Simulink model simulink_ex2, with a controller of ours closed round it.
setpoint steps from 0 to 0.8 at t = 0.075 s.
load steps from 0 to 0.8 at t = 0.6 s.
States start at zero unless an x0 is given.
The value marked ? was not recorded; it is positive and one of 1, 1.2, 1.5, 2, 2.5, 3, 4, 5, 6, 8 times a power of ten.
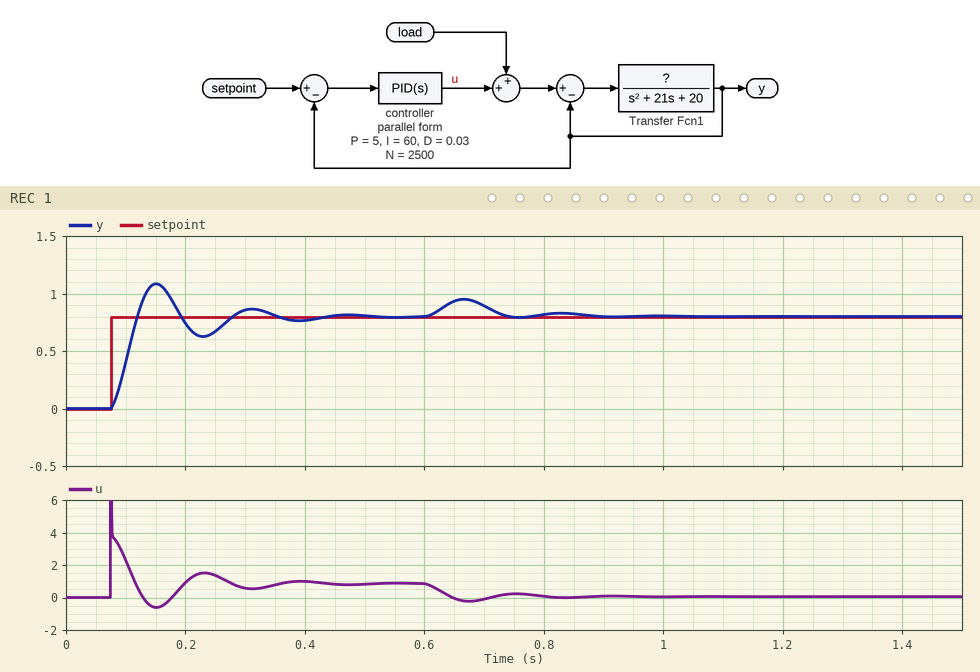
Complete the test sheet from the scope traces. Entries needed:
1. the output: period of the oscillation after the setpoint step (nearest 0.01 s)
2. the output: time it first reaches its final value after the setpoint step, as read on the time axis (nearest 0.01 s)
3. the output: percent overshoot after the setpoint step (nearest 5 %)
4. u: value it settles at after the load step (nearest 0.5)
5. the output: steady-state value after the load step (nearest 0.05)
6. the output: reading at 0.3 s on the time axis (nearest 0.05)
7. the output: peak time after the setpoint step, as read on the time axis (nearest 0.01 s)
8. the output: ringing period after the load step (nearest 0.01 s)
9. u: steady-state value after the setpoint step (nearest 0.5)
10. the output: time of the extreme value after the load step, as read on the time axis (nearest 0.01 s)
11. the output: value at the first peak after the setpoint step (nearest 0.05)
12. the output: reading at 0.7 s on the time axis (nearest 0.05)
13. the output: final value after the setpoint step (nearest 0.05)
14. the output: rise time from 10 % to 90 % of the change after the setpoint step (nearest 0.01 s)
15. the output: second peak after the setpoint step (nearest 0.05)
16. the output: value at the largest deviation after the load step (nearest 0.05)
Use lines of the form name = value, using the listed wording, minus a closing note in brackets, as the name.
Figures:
the output: period of the oscillation after the setpoint step = 0.16 s
the output: time it first reaches its final value after the setpoint step, as read on the time axis = 0.12 s
the output: percent overshoot after the setpoint step = 35 %
u: value it settles at after the load step = 0.0
the output: steady-state value after the load step = 0.80
the output: reading at 0.3 s on the time axis = 0.85
the output: peak time after the setpoint step, as read on the time axis = 0.15 s
the output: ringing period after the load step = 0.16 s
u: steady-state value after the setpoint step = 1.0
the output: time of the extreme value after the load step, as read on the time axis = 0.67 s
the output: value at the first peak after the setpoint step = 1.10
the output: reading at 0.7 s on the time axis = 0.90
the output: final value after the setpoint step = 0.80
the output: rise time from 10 % to 90 % of the change after the setpoint step = 0.03 s
the output: second peak after the setpoint step = 0.85
the output: value at the largest deviation after the load step = 0.95
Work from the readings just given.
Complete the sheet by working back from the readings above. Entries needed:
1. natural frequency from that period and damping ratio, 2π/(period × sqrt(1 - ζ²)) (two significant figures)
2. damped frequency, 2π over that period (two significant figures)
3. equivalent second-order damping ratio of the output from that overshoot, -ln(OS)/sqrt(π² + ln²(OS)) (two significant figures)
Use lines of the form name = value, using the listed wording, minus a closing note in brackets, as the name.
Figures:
natural frequency from that period and damping ratio, 2π/(period × sqrt(1 - ζ²)) = 41 rad/s
damped frequency, 2π over that period = 39 rad/s
equivalent second-order damping ratio of the output from that overshoot, -ln(OS)/sqrt(π² + ln²(OS)) = 0.32
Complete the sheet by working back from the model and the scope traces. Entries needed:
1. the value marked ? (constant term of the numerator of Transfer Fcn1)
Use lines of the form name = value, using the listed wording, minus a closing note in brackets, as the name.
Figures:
the value marked ? = 300
